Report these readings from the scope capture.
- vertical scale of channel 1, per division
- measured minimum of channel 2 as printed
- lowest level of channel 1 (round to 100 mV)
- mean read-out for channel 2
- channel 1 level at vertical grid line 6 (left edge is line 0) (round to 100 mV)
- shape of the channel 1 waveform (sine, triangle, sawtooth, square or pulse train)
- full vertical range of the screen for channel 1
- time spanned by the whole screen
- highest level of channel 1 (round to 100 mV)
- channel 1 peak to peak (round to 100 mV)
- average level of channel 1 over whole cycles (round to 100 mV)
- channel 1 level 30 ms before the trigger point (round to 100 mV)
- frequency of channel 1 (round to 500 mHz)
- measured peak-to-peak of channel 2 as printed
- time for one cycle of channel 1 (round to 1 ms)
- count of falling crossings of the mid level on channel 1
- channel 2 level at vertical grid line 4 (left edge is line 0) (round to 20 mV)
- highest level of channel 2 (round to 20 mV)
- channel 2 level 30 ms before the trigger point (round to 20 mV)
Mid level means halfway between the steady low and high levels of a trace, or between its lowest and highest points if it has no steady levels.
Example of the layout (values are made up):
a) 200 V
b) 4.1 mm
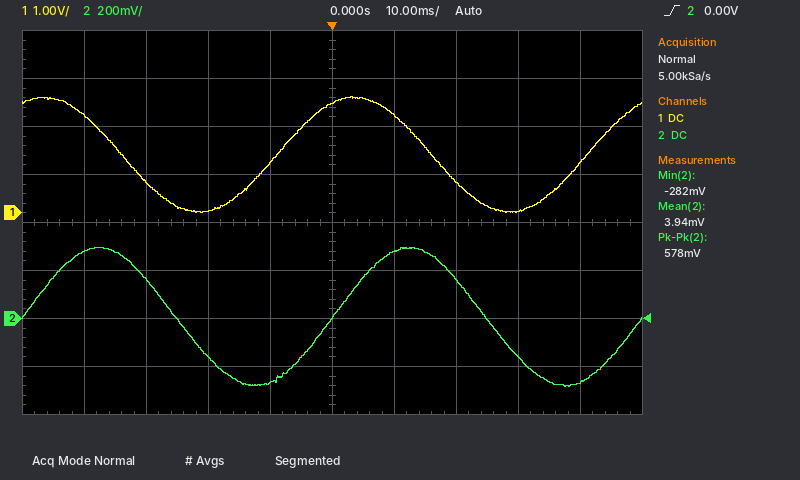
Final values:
a) 1 V
b) -282 mV
c) 0.0 V
d) 3.94 mV
e) 2.0 V
f) sine
g) 8 V
h) 100 ms
i) 2.4 V
j) 2.4 V
k) 1.2 V
l) 600 mV
m) 20.0 Hz
n) 578 mV
o) 50 ms
p) 2
q) -260 mV
r) 300 mV
s) 160 mV
